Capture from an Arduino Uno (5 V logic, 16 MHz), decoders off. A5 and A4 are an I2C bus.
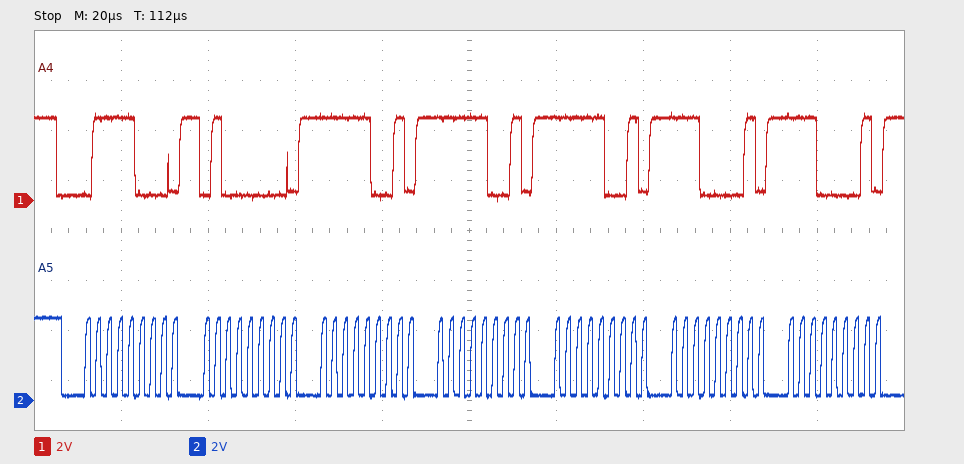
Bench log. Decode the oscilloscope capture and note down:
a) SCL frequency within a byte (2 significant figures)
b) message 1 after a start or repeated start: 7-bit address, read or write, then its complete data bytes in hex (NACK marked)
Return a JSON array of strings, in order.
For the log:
["400 kHz", "0x3C write: 40 F9 F9 F9 E1 E1"]
